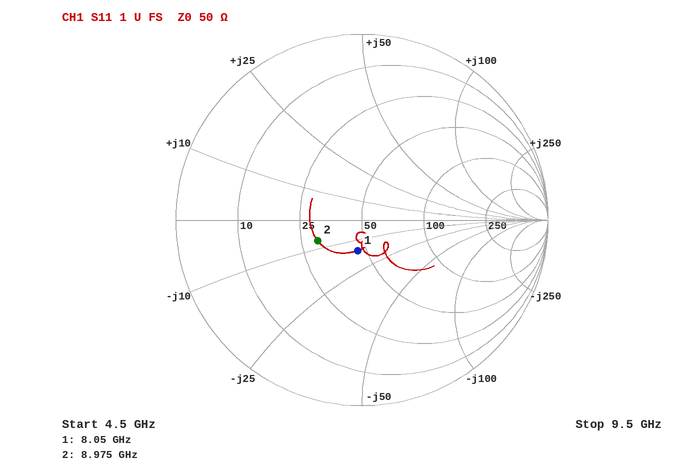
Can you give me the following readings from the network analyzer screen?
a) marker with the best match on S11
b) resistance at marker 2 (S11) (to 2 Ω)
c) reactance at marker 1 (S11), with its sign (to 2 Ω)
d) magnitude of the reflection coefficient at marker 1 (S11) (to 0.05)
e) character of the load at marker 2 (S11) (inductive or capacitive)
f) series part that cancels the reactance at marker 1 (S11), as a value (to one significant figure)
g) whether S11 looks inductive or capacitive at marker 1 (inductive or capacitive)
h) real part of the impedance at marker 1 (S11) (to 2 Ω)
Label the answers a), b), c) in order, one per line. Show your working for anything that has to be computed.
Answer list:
a) marker 1
b) 30 Ω
c) -16 Ω
d) 0.15
e) capacitive
f) L = 16 Ω/(2π × 8.05 GHz) ≈ 316 pH, so 300 pH to one significant figure
g) capacitive
h) 46 Ω
